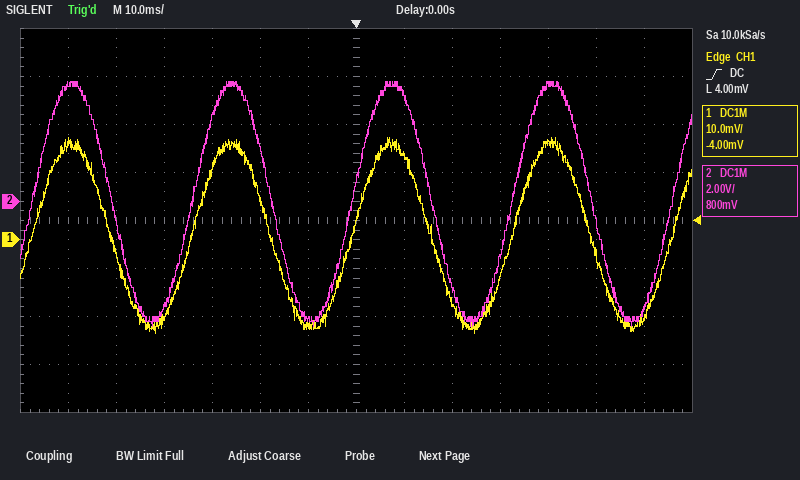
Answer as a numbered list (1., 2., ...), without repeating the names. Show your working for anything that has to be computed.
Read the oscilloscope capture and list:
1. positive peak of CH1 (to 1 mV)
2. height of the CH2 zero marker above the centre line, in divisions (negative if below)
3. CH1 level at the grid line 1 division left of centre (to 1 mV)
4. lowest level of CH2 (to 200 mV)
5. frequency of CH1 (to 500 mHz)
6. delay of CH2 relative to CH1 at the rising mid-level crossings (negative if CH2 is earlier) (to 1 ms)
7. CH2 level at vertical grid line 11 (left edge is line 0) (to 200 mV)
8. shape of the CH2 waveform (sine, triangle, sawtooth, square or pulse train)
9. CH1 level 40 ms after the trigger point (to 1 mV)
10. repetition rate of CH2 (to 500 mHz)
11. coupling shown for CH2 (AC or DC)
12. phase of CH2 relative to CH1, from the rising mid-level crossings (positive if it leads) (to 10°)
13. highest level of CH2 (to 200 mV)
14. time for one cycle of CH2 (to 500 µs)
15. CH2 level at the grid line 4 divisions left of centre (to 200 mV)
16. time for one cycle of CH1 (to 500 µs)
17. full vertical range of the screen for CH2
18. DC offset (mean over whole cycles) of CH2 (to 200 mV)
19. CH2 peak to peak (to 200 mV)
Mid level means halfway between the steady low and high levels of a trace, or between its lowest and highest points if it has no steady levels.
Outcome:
1. 21 mV
2. +0.4 div
3. -18 mV
4. -5.2 V
5. 1 / 33.5 ms ≈ 29.9 Hz, so 30.0 Hz to the nearest 500 mHz
6. 0 ms
7. 4.8 V
8. sine
9. 20 mV
10. 1 / 33.5 ms ≈ 29.9 Hz, so 30.0 Hz to the nearest 500 mHz
11. DC
12. −360° × (0 ms) / 33.5 ms ≈ 0°
13. 5.0 V
14. 33.5 ms
15. -4.4 V
16. 33.5 ms
17. 16 V
18. (5.0 V + (-5.2 V)) / 2 ≈ 0.0 V
19. 5.0 V − (-5.2 V) = 10.2 V
